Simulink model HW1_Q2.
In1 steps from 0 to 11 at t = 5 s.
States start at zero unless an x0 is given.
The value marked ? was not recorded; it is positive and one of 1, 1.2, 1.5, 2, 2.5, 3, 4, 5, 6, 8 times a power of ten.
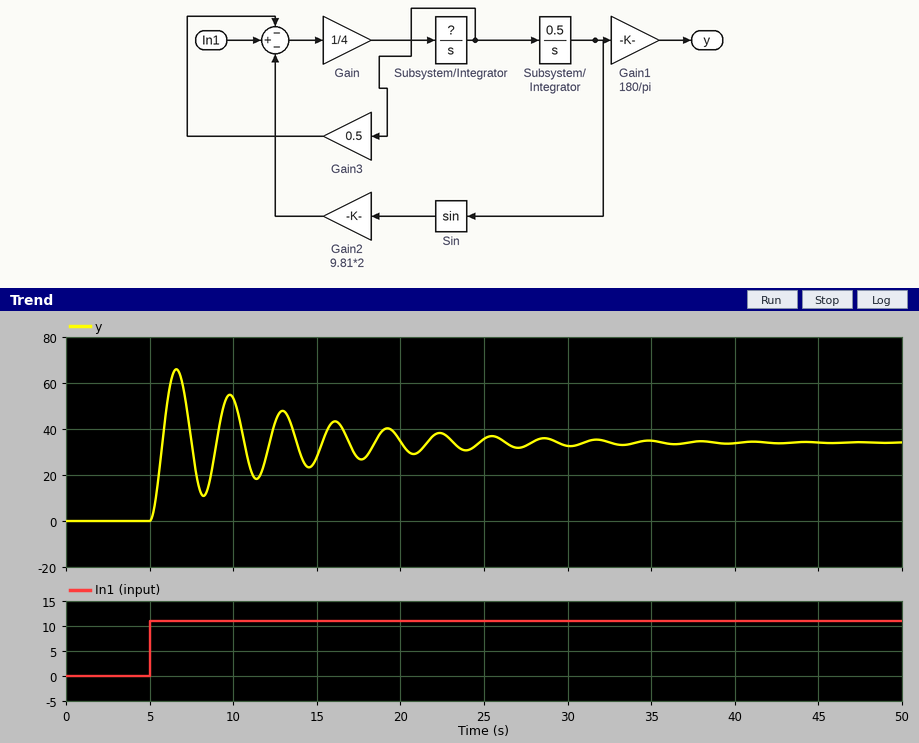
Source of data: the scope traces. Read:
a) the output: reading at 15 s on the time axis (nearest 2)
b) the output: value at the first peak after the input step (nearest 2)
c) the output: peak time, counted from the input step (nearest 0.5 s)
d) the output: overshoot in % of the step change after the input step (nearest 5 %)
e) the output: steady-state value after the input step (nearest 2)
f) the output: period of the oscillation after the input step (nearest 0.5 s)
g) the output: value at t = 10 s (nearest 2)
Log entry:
28
66
1.5 s
95 %
34
3.0 s
54
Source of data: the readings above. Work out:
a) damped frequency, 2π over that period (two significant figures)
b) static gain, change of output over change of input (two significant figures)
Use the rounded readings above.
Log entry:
2.1 rad/s
3.1
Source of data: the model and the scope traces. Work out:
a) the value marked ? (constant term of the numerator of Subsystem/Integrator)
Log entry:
2
